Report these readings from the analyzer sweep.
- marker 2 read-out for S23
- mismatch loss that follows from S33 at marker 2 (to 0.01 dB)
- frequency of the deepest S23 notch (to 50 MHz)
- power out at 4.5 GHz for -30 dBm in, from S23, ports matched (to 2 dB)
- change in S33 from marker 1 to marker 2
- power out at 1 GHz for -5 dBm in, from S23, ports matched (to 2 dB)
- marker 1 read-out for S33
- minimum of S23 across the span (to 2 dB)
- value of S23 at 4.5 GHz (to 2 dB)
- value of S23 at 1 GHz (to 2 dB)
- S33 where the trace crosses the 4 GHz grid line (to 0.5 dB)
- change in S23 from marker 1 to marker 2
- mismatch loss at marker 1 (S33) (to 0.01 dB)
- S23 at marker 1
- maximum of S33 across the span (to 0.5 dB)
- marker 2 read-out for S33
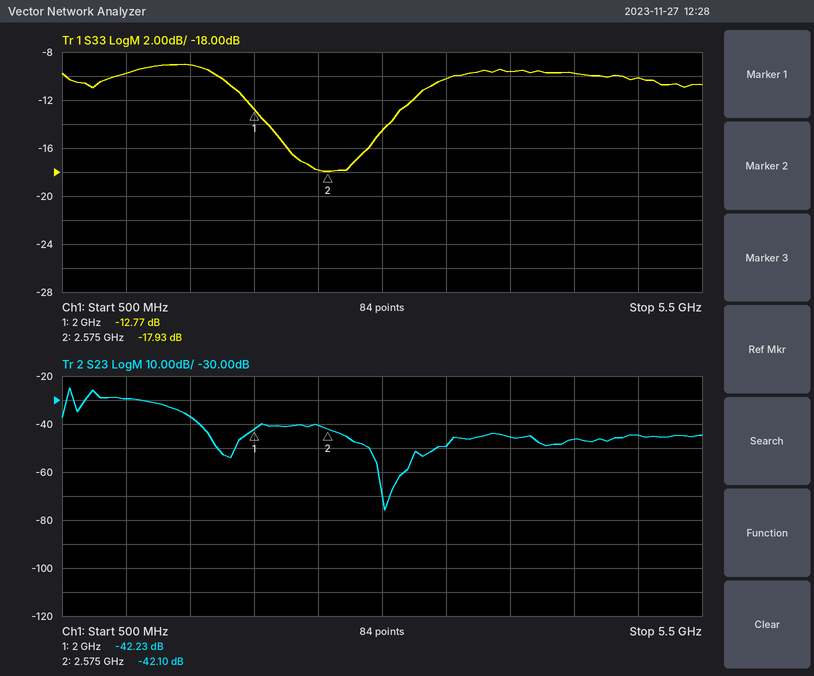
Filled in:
-42.10 dB
0.07 dB
3.00 GHz
-76 dBm
-5.16 dB
-34 dBm
-12.77 dB
-76 dB
-46 dB
-30 dB
-9.5 dB
0.13 dB
0.24 dB
-42.23 dB
-9.0 dB
-17.93 dB
